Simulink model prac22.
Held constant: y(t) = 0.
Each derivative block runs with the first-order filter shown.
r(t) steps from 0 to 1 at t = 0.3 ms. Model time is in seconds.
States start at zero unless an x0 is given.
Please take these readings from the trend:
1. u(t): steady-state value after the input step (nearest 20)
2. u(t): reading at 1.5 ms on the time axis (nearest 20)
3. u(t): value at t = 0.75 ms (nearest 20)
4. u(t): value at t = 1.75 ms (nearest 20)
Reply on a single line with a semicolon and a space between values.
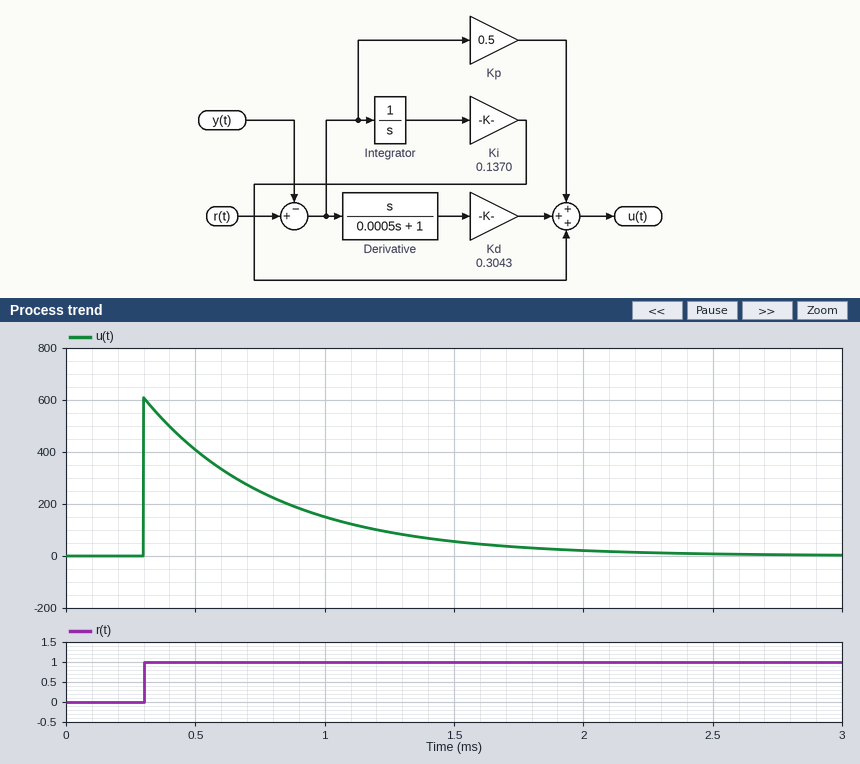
0; 60; 240; 40
